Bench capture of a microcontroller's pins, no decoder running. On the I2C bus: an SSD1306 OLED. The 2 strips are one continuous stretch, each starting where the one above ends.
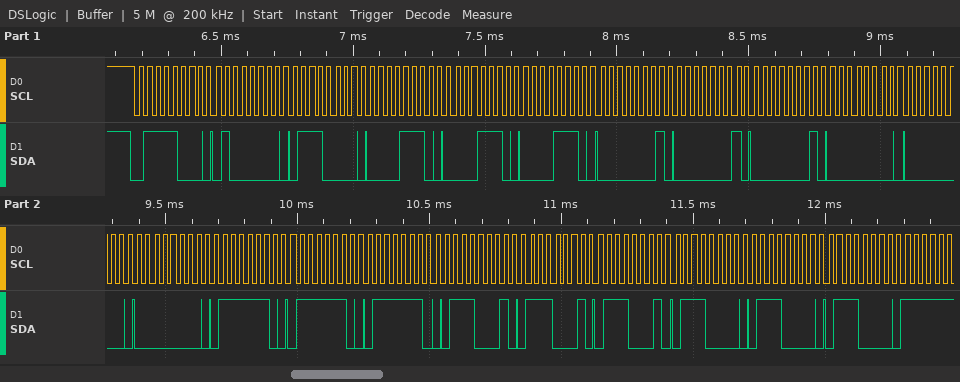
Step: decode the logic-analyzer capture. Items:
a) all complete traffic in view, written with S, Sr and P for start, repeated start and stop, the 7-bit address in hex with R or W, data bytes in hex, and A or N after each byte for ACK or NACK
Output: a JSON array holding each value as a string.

["S 3CW A 40 A 70 A 0E A 0E A 0E A 01 A 01 A 01 A 00 A 00 A 00 A 7E A 7E A 7E A 71 A 71 A 71 A 70 A 70 A 70 A"]
